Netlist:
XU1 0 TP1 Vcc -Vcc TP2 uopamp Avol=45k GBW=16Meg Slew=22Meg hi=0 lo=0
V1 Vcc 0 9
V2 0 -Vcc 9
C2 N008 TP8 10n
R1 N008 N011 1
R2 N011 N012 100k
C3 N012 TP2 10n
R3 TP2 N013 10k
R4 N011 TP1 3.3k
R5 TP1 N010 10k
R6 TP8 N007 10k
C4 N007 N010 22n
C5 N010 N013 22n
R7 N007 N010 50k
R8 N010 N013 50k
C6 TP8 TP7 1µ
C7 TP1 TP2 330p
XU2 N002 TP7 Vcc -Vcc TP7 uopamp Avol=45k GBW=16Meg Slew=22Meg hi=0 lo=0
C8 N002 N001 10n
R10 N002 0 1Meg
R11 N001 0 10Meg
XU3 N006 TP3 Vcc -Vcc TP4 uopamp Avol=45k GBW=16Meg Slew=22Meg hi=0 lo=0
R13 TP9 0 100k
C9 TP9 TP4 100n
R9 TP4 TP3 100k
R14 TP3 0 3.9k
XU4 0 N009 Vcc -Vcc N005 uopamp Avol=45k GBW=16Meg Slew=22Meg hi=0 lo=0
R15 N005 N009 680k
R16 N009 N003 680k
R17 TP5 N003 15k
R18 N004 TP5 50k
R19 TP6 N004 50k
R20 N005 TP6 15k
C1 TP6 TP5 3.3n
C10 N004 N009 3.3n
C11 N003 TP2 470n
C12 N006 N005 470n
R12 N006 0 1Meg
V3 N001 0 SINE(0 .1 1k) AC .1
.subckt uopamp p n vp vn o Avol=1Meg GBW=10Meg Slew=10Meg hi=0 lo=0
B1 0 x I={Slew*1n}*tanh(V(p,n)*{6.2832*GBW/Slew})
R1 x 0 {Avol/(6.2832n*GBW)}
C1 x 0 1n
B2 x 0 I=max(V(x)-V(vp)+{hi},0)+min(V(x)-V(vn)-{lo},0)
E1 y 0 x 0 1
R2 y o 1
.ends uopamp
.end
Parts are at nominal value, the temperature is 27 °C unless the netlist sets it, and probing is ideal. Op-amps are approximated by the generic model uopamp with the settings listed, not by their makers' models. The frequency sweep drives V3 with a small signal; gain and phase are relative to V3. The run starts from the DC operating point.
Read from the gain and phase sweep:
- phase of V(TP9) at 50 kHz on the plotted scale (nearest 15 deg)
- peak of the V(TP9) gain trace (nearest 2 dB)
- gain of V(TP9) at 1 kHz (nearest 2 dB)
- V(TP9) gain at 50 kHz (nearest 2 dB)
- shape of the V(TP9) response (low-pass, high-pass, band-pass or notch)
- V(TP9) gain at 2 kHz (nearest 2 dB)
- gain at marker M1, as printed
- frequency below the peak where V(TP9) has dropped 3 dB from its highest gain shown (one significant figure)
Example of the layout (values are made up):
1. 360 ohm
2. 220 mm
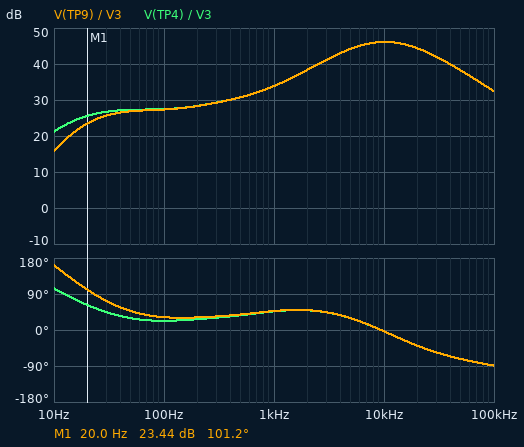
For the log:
1. -75 deg
2. 46 dB
3. 34 dB
4. 38 dB
5. band-pass
6. 38 dB
7. 23.44 dB
8. 4 kHz
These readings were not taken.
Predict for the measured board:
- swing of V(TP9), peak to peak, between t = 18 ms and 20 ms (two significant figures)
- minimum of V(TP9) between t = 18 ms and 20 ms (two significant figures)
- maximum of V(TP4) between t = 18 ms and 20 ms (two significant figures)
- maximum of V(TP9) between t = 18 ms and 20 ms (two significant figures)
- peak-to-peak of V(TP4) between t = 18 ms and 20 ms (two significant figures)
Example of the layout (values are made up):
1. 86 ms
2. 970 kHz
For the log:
1. 9.9 V
2. -4.9 V
3. 4.9 V
4. 4.9 V
5. 9.9 V
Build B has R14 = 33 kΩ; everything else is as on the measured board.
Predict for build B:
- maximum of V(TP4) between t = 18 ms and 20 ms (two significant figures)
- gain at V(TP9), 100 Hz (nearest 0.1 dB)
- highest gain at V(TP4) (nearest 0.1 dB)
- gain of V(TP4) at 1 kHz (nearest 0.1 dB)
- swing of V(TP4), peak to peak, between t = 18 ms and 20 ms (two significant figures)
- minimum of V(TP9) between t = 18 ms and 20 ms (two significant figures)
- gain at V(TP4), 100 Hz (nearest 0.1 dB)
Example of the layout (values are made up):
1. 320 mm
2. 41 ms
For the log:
1. 750 mV
2. 11.0 dB
3. 29.7 dB
4. 17.5 dB
5. 1.5 V
6. -750 mV
7. 11.1 dB
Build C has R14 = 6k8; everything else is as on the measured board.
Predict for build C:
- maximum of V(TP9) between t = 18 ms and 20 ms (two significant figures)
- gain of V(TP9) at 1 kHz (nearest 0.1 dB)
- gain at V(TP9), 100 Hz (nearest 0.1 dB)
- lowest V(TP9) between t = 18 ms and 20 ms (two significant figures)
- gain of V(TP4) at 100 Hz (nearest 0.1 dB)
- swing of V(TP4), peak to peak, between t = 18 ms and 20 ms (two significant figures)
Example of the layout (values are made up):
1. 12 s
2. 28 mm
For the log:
1. 2.9 V
2. 29.3 dB
3. 22.8 dB
4. -2.9 V
5. 22.9 dB
6. 5.8 V
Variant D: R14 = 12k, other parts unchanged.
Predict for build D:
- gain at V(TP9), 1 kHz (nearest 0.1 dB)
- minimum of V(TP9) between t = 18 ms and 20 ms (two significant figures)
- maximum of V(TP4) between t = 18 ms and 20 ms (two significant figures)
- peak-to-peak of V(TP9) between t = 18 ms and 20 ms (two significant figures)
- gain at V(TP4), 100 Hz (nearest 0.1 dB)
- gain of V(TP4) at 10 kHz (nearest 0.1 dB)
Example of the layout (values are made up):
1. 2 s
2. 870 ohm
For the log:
1. 24.8 dB
2. -1.7 V
3. 1.7 V
4. 3.5 V
5. 18.4 dB
6. 37.0 dB
